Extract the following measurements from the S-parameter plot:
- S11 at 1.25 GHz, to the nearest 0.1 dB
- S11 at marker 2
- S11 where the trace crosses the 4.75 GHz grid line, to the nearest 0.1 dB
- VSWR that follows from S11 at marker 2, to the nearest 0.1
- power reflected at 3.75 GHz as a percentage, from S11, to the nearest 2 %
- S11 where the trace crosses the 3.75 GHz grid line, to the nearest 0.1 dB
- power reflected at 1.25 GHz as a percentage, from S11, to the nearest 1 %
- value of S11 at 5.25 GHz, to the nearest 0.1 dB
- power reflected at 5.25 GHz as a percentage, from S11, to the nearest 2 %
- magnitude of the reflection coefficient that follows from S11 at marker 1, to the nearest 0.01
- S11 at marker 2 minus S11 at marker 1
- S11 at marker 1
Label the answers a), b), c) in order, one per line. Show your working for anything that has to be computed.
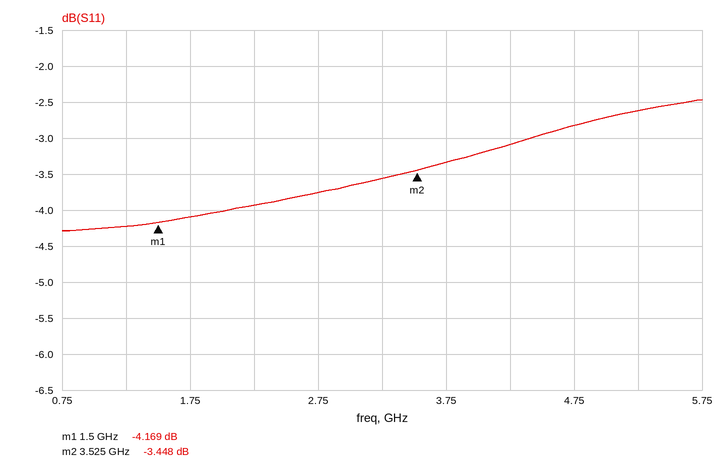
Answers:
a) -4.2 dB
b) -3.448 dB
c) -2.8 dB
d) (1 + 0.6724)/(1 − 0.6724) ≈ 5.1
e) 10^(-3.3/10) ≈ 46.8 %, so 46 % to the nearest 2 %
f) -3.3 dB
g) 10^(-4.2/10) ≈ 38 %
h) -2.6 dB
i) 10^(-2.6/10) ≈ 55.0 %, so 54 % to the nearest 2 %
j) 10^(-4.169/20) ≈ 0.62
k) -3.448 − (-4.169) = 0.721 dB
l) -4.169 dB
